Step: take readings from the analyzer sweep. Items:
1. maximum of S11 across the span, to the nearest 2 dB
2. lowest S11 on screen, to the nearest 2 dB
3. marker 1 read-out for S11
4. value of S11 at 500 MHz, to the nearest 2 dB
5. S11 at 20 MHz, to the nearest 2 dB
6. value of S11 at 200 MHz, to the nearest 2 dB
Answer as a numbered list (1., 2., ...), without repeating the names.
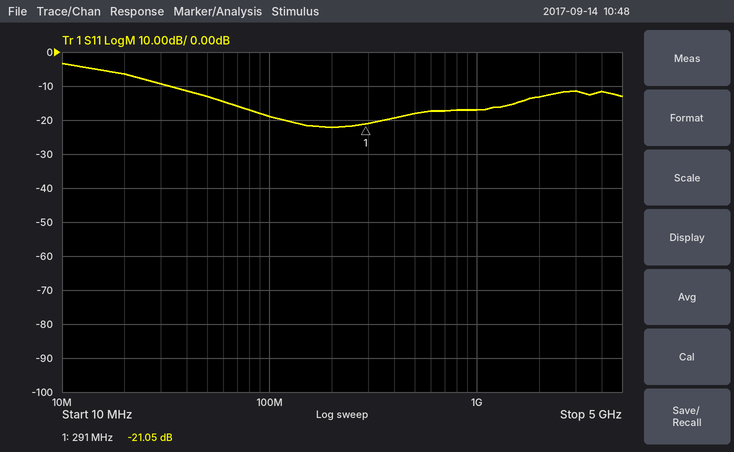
1. -4 dB
2. -22 dB
3. -21.05 dB
4. -18 dB
5. -6 dB
6. -22 dB
